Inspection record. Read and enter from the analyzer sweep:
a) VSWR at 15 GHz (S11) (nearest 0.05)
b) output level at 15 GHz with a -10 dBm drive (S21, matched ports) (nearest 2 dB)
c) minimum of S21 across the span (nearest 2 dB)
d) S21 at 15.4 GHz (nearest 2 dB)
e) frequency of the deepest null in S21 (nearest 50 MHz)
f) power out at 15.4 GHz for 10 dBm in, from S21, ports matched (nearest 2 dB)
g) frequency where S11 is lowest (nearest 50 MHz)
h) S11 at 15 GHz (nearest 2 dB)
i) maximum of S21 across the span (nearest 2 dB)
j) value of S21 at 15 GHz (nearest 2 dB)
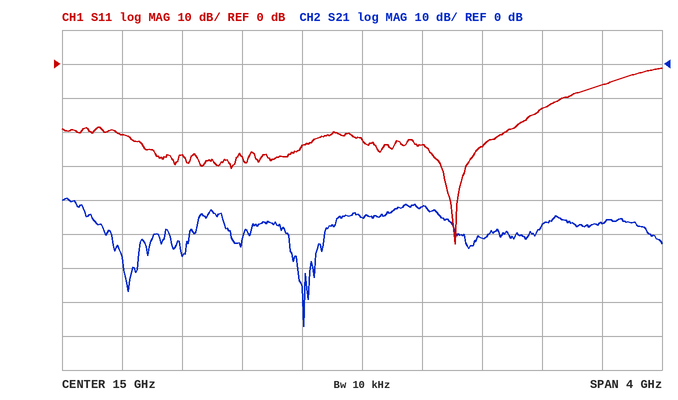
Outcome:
1.15
-56 dBm
-78 dB
-42 dB
14.60 GHz
-32 dBm
15.60 GHz
-22 dB
-40 dB
-46 dB
